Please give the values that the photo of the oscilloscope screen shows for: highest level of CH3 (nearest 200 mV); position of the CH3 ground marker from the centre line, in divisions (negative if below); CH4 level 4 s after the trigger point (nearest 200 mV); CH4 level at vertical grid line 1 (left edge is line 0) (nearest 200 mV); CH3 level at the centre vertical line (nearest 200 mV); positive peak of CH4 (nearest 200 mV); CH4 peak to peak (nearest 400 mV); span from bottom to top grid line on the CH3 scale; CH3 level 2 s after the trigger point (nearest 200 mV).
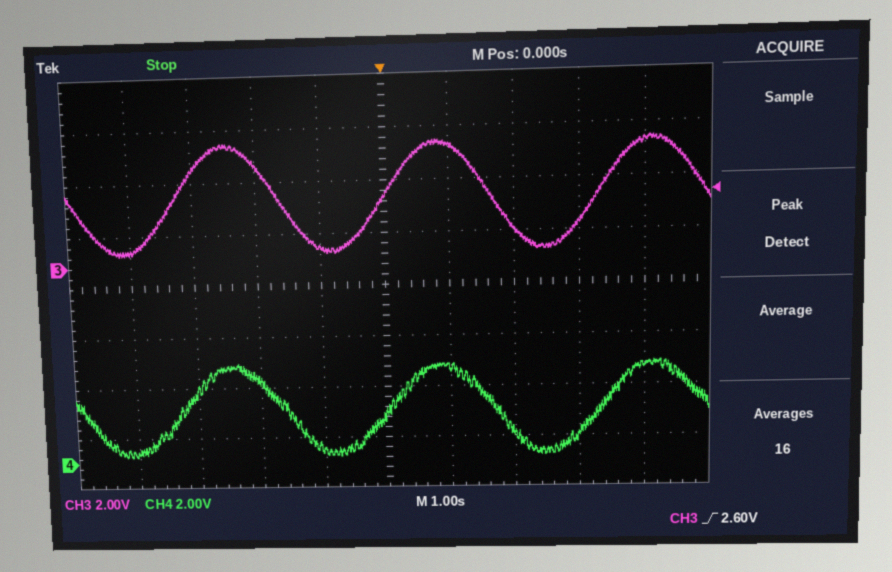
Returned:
4.6 V
+0.4 div
3.8 V
400 mV
2.6 V
4.0 V
3.6 V
16 V
1.2 V
